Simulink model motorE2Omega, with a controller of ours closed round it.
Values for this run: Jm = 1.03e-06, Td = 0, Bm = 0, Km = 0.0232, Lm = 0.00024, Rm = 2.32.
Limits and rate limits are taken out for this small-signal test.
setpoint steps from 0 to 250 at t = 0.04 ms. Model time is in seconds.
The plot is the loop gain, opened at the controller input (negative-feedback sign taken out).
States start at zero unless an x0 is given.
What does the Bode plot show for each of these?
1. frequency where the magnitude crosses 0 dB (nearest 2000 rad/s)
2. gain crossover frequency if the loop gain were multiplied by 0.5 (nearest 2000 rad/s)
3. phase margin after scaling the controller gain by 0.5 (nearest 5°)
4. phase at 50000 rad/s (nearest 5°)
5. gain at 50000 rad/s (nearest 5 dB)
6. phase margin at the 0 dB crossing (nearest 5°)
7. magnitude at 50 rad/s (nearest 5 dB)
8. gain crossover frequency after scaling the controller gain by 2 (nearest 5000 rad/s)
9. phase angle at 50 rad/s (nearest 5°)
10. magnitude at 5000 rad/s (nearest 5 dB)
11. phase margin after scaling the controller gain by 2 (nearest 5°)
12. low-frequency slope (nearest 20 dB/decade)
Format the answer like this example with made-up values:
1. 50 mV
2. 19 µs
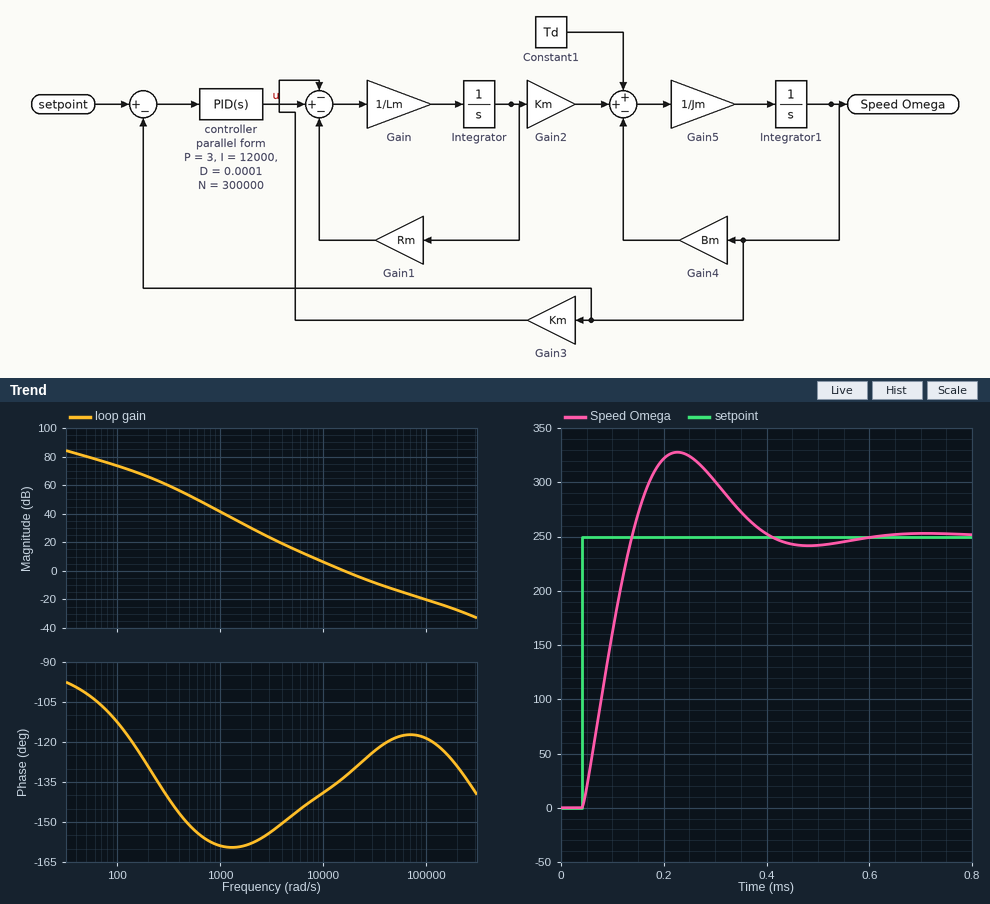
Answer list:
1. 16000 rad/s
2. 10000 rad/s
3. 40°
4. -120°
5. -15 dB
6. 45°
7. 80 dB
8. 25000 rad/s
9. -100°
10. 15 dB
11. 55°
12. -20 dB/decade
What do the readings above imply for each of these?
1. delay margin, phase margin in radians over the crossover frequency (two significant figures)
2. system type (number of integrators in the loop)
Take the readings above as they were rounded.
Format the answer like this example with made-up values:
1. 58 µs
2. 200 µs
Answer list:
1. 0.000049 s
2. 1
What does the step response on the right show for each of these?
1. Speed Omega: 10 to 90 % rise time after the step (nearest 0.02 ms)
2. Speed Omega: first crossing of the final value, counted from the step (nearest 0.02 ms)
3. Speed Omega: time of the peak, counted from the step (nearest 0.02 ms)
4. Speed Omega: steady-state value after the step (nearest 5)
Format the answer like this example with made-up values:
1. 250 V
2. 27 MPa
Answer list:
1. 0.08 ms
2. 0.10 ms
3. 0.18 ms
4. 250
